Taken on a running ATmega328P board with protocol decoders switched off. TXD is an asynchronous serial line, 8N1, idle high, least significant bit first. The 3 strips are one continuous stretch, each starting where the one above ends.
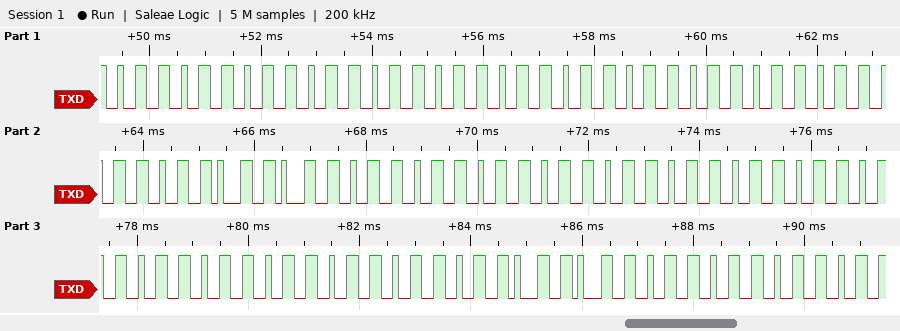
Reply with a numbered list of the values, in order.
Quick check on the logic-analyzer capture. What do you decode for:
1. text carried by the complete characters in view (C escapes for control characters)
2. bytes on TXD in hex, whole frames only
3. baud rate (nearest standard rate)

1. "2222222222222211222222222222222112222"
2. 0x32 0x32 0x32 0x32 0x32 0x32 0x32 0x32 0x32 0x32 0x32 0x32 0x32 0x32 0x31 0x31 0x32 0x32 0x32 0x32 0x32 0x32 0x32 0x32 0x32 0x32 0x32 0x32 0x32 0x32 0x32 0x31 0x31 0x32 0x32 0x32 0x32
3. 9600 baud
